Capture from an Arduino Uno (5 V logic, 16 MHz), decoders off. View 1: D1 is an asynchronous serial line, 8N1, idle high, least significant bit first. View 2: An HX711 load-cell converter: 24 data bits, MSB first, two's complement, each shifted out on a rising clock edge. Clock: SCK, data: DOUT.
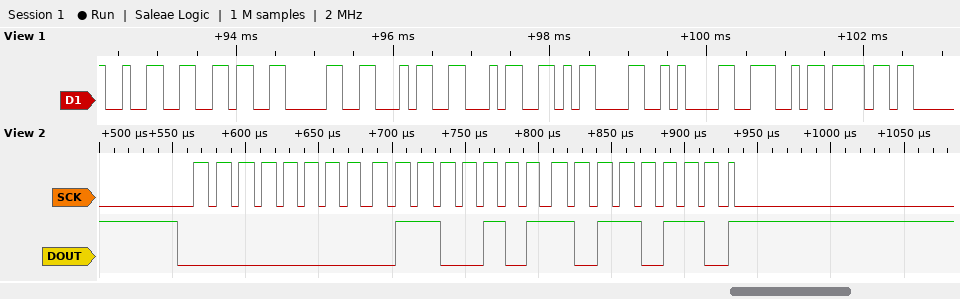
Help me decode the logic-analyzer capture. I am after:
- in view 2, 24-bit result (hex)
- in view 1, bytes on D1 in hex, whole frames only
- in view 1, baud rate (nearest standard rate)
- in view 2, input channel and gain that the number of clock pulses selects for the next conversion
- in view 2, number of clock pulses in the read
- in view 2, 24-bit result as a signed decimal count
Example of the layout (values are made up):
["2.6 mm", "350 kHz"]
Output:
["0x0065B6", "32 36 30 34 34 0D 0A 4E 6F", "9600 baud", "channel A, gain 128", "25", "26038"]
